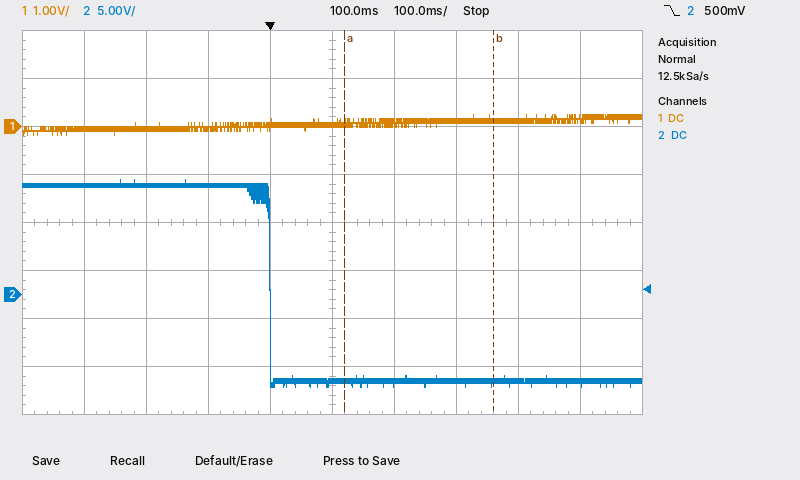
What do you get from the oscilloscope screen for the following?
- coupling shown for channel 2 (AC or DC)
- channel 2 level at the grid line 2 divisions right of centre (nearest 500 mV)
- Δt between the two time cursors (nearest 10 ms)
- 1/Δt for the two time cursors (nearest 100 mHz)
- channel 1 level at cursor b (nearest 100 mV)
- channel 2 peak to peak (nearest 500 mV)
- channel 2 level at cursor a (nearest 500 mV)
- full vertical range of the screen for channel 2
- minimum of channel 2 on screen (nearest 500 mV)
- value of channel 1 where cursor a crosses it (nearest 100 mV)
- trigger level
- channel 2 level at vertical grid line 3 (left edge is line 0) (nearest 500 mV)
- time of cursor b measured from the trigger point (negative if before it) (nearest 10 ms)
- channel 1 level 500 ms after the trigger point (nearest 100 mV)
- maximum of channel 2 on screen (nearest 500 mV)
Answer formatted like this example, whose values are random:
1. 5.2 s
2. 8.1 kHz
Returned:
1. DC
2. -9.0 V
3. 240 ms
4. 4.2 Hz
5. 100 mV
6. 21.5 V
7. -9.0 V
8. 40 V
9. -9.5 V
10. 100 mV
11. 500 mV
12. 11.5 V
13. +360 ms
14. 200 mV
15. 12.0 V
